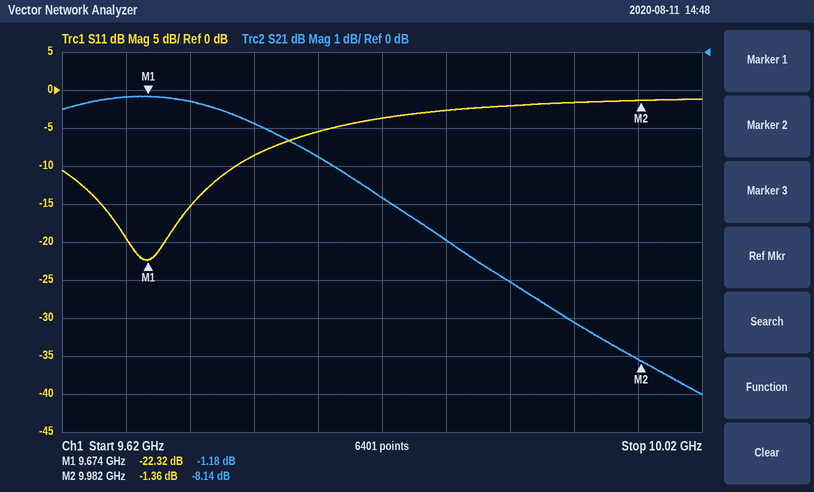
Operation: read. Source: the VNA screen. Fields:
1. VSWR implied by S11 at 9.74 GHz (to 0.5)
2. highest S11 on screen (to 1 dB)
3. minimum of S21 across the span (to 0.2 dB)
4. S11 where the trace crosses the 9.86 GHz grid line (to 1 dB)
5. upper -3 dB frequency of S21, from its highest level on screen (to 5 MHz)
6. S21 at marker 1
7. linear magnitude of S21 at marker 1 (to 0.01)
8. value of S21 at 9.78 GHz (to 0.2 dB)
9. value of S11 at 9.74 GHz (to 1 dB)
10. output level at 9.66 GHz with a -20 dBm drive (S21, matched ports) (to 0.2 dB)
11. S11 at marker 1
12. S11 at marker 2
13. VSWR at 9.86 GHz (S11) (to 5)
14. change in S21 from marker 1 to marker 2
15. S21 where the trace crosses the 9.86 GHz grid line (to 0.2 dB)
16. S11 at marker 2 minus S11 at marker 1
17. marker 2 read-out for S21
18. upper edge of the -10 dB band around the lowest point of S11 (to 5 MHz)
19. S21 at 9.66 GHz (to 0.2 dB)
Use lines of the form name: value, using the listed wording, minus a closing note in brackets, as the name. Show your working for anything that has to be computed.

VSWR implied by S11 at 9.74 GHz: |Γ| = 10^(-9/20) = 0.3548; VSWR = (1 + 0.3548)/(1 − 0.3548) ≈ 2.10, so 2.0 to the nearest 0.5
highest S11 on screen: -1 dB
minimum of S21 across the span: -9.0 dB
S11 where the trace crosses the 9.86 GHz grid line: -3 dB
upper -3 dB frequency of S21, from its highest level on screen: 9.830 GHz
S21 at marker 1: -1.18 dB
linear magnitude of S21 at marker 1: 10^(-1.18/20) ≈ 0.87
value of S21 at 9.78 GHz: -2.8 dB
value of S11 at 9.74 GHz: -9 dB
output level at 9.66 GHz with a -20 dBm drive (S21, matched ports): -20 dBm + (-1.2 dB) = -21.2 dBm
S11 at marker 1: -22.32 dB
S11 at marker 2: -1.36 dB
VSWR at 9.86 GHz (S11): |Γ| = 10^(-3/20) = 0.7079; VSWR = (1 + 0.7079)/(1 − 0.7079) ≈ 5.85, so 5 to the nearest 5
change in S21 from marker 1 to marker 2: -8.14 − (-1.18) = -6.96 dB
S21 where the trace crosses the 9.86 GHz grid line: -5.0 dB
S11 at marker 2 minus S11 at marker 1: -1.36 − (-22.32) = 20.96 dB
marker 2 read-out for S21: -8.14 dB
upper edge of the -10 dB band around the lowest point of S11: 9.730 GHz
S21 at 9.66 GHz: -1.2 dB
